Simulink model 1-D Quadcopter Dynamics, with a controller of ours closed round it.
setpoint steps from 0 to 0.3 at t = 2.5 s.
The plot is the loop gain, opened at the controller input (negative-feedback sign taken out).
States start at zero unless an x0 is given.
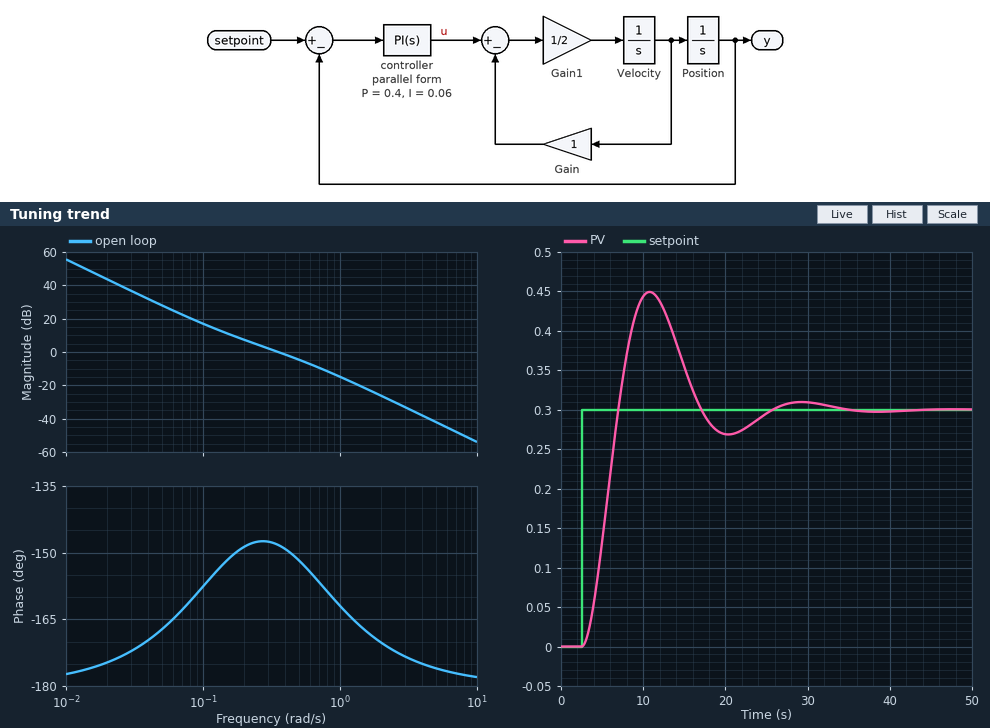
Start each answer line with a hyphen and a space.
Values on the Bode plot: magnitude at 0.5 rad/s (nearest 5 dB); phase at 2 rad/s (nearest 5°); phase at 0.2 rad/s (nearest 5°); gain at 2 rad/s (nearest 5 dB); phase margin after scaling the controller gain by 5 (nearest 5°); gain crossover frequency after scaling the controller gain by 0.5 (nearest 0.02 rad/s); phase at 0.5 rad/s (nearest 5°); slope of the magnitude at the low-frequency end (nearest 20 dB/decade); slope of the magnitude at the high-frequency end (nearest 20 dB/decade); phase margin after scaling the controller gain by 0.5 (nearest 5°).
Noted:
- -5 dB
- -170°
- -150°
- -25 dB
- 20°
- 0.22 rad/s
- -150°
- -40 dB/decade
- -40 dB/decade
- 30°
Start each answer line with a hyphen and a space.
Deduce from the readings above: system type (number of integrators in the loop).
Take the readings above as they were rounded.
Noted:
- 2
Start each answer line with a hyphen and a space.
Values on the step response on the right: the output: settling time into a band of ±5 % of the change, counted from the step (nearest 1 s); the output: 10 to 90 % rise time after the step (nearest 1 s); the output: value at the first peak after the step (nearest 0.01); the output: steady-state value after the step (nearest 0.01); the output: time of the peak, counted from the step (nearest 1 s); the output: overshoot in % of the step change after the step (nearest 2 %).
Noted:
- 21 s
- 3 s
- 0.45
- 0.30
- 8 s
- 50 %
